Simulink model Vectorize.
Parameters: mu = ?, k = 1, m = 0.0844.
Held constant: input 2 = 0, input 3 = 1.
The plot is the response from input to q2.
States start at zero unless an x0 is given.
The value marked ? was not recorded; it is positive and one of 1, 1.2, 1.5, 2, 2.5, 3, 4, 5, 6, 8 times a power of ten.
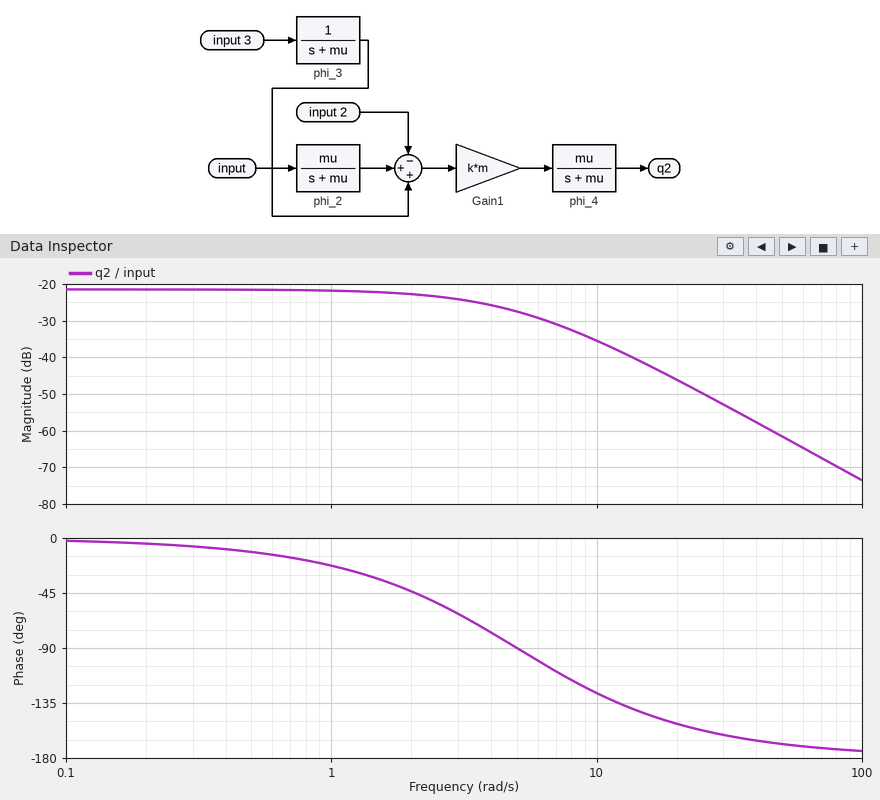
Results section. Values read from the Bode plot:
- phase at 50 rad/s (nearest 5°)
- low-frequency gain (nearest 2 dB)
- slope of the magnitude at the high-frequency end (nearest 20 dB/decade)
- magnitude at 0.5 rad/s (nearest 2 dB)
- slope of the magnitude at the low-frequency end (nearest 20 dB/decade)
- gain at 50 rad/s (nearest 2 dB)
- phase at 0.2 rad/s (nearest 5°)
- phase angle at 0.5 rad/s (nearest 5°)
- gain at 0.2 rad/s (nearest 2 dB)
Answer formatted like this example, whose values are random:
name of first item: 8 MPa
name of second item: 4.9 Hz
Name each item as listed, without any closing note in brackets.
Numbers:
phase at 50 rad/s: -170°
low-frequency gain: -22 dB
slope of the magnitude at the high-frequency end: -40 dB/decade
magnitude at 0.5 rad/s: -22 dB
slope of the magnitude at the low-frequency end: 0 dB/decade
gain at 50 rad/s: -62 dB
phase at 0.2 rad/s: -5°
phase angle at 0.5 rad/s: -10°
gain at 0.2 rad/s: -22 dB
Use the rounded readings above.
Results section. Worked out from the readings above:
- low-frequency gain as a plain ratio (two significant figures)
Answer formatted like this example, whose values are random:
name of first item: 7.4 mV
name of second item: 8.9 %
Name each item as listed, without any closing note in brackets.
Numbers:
low-frequency gain as a plain ratio: 0.079
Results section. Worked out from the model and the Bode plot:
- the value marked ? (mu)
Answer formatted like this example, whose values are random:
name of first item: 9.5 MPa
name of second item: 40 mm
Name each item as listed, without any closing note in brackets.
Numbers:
the value marked ?: 5
